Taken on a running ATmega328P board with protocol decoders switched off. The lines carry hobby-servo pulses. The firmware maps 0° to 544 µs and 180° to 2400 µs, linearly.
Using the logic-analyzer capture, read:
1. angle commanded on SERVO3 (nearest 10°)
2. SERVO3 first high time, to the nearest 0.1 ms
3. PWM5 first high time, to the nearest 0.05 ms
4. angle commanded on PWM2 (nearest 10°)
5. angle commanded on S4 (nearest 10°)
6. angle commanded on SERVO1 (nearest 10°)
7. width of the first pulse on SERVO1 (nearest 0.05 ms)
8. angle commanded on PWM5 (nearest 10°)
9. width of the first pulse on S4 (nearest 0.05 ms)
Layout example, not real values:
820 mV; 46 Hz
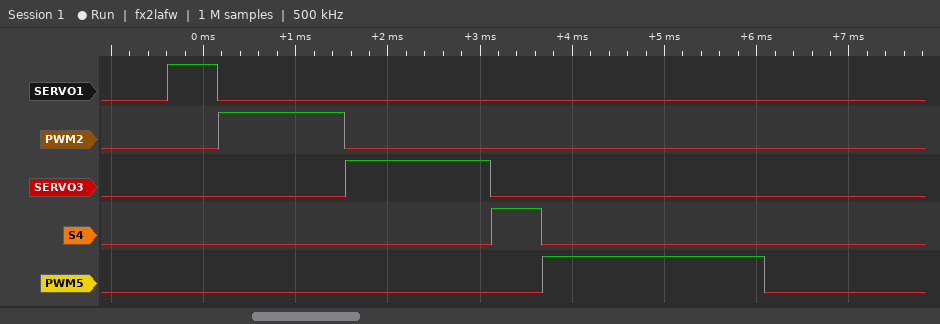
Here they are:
100°; 1.6 ms; 2.40 ms; 80°; 0°; 0°; 0.55 ms; 180°; 0.55 ms
